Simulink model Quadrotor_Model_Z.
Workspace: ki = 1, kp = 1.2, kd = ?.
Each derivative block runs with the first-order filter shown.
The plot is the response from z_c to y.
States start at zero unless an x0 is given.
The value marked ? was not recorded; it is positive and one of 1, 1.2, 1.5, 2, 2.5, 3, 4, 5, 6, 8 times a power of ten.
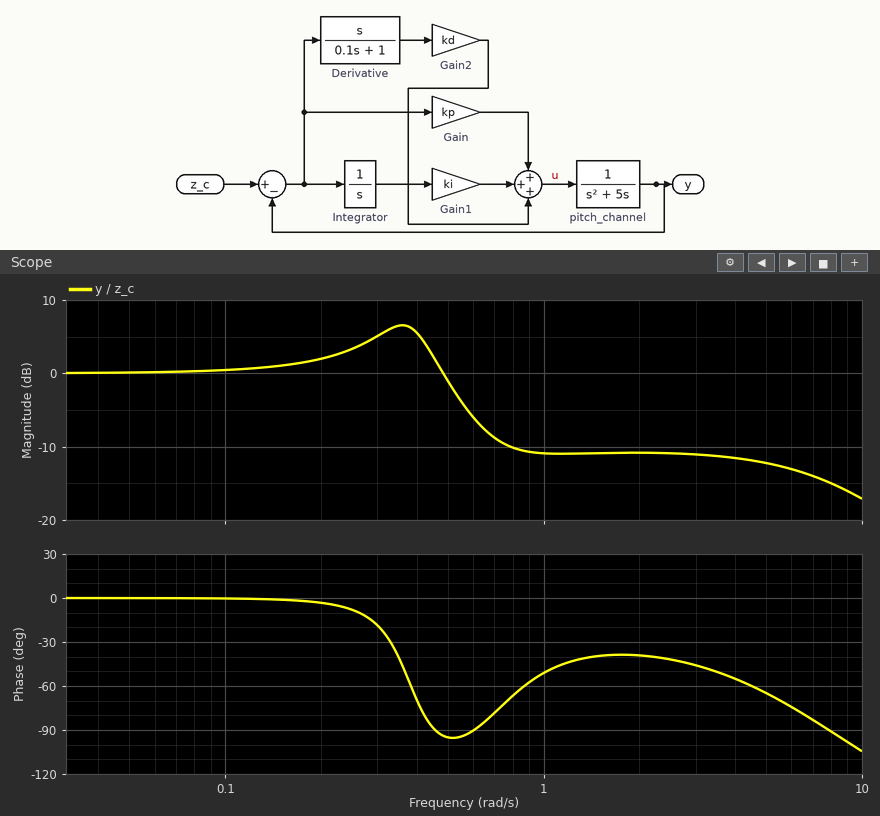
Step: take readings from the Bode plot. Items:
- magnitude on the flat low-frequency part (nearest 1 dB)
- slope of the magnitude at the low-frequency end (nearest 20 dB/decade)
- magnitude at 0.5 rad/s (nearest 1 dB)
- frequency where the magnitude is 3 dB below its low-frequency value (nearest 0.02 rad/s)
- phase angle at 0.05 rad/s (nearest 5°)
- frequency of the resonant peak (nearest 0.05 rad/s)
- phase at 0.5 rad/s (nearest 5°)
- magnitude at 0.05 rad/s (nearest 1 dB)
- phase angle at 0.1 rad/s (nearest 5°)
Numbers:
0 dB
0 dB/decade
-1 dB
0.54 rad/s
0°
0.35 rad/s
-95°
0 dB
0°
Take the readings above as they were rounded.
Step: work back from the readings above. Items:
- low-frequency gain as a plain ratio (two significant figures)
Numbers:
1.0
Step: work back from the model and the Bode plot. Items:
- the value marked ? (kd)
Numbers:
2
